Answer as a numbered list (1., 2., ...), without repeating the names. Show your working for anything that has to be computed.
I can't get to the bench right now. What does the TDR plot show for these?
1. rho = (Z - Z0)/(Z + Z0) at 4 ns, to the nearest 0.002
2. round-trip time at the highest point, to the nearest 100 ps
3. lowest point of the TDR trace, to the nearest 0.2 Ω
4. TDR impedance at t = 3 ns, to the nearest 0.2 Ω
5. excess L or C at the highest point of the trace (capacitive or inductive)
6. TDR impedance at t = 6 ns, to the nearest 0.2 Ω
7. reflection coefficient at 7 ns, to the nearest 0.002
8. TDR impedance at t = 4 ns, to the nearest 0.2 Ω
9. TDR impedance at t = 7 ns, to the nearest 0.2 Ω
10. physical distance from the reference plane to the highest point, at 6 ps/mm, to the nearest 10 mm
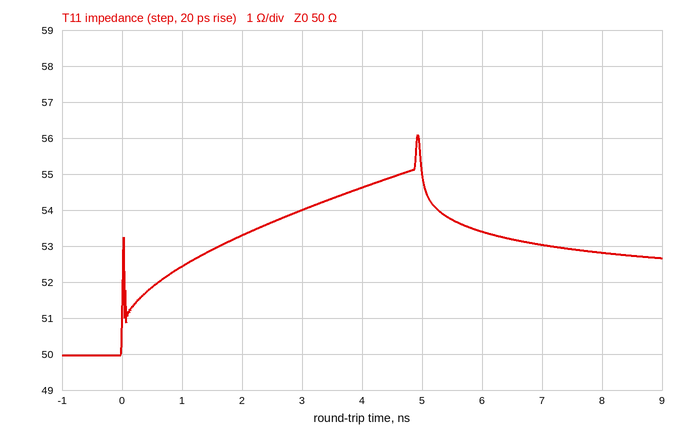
1. (54.6 − 50)/(54.6 + 50) ≈ +0.044
2. 4.9 ns
3. 50.0 Ω
4. 54.0 Ω
5. inductive
6. 53.4 Ω
7. (53 − 50)/(53 + 50) ≈ +0.0291, so +0.030 to the nearest 0.002
8. 54.6 Ω
9. 53.0 Ω
10. 4.9 ns / 2 / 6 ps/mm ≈ 408 mm, so 410 mm to the nearest 10 mm
